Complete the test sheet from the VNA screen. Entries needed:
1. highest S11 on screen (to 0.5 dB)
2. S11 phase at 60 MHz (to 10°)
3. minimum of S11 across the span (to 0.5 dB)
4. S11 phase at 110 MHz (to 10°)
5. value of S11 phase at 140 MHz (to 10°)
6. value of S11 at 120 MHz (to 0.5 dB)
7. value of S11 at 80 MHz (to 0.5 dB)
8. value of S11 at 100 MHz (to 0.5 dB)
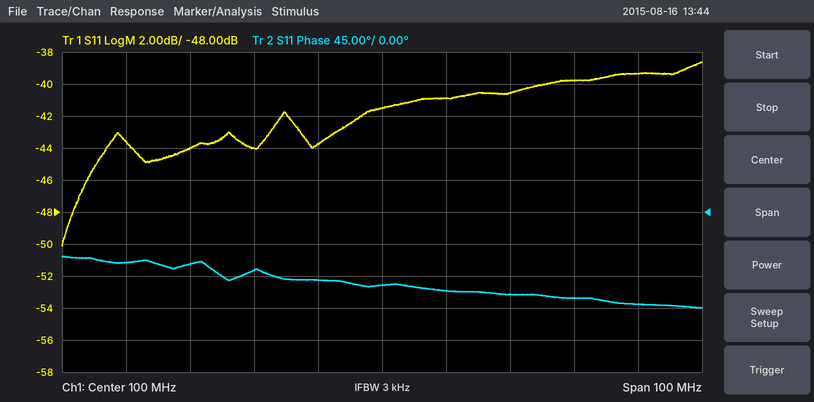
-38.5 dB
-70°
-50.0 dB
-110°
-130°
-40.5 dB
-44.0 dB
-41.5 dB
